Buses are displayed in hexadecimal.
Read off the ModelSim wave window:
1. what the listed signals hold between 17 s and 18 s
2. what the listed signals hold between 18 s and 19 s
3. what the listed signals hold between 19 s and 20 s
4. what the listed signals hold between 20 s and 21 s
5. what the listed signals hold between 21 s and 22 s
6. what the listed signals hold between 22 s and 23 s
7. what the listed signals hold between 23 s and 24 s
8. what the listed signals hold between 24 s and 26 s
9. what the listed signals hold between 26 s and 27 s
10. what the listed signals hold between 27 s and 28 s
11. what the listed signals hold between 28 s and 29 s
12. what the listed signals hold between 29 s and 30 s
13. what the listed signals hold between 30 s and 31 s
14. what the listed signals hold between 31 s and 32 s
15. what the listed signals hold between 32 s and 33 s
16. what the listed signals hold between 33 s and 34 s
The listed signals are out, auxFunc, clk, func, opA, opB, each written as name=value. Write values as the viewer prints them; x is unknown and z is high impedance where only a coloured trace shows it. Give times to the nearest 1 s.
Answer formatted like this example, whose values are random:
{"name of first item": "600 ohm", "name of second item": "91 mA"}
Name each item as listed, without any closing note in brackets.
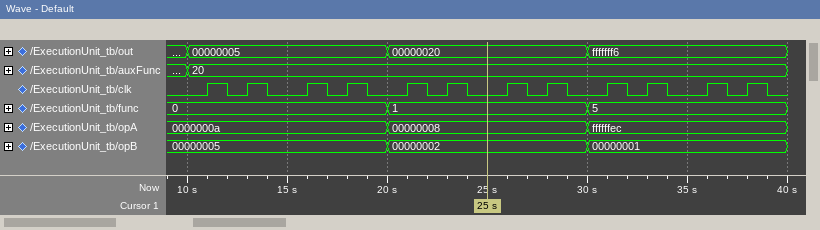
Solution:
{"what the listed signals hold between 17 s and 18 s": "out=00000005, auxFunc=20, clk=0, func=0, opA=0000000a, opB=00000005", "what the listed signals hold between 18 s and 19 s": "out=00000005, auxFunc=20, clk=1, func=0, opA=0000000a, opB=00000005", "what the listed signals hold between 19 s and 20 s": "out=00000005, auxFunc=20, clk=0, func=0, opA=0000000a, opB=00000005", "what the listed signals hold between 20 s and 21 s": "out=00000020, auxFunc=20, clk=0, func=1, opA=00000008, opB=00000002", "what the listed signals hold between 21 s and 22 s": "out=00000020, auxFunc=20, clk=1, func=1, opA=00000008, opB=00000002", "what the listed signals hold between 22 s and 23 s": "out=00000020, auxFunc=20, clk=0, func=1, opA=00000008, opB=00000002", "what the listed signals hold between 23 s and 24 s": "out=00000020, auxFunc=20, clk=1, func=1, opA=00000008, opB=00000002", "what the listed signals hold between 24 s and 26 s": "out=00000020, auxFunc=20, clk=0, func=1, opA=00000008, opB=00000002", "what the listed signals hold between 26 s and 27 s": "out=00000020, auxFunc=20, clk=1, func=1, opA=00000008, opB=00000002", "what the listed signals hold between 27 s and 28 s": "out=00000020, auxFunc=20, clk=0, func=1, opA=00000008, opB=00000002", "what the listed signals hold between 28 s and 29 s": "out=00000020, auxFunc=20, clk=1, func=1, opA=00000008, opB=00000002", "what the listed signals hold between 29 s and 30 s": "out=00000020, auxFunc=20, clk=0, func=1, opA=00000008, opB=00000002", "what the listed signals hold between 30 s and 31 s": "out=fffffff6, auxFunc=20, clk=0, func=5, opA=ffffffec, opB=00000001", "what the listed signals hold between 31 s and 32 s": "out=fffffff6, auxFunc=20, clk=1, func=5, opA=ffffffec, opB=00000001", "what the listed signals hold between 32 s and 33 s": "out=fffffff6, auxFunc=20, clk=0, func=5, opA=ffffffec, opB=00000001", "what the listed signals hold between 33 s and 34 s": "out=fffffff6, auxFunc=20, clk=1, func=5, opA=ffffffec, opB=00000001"}
